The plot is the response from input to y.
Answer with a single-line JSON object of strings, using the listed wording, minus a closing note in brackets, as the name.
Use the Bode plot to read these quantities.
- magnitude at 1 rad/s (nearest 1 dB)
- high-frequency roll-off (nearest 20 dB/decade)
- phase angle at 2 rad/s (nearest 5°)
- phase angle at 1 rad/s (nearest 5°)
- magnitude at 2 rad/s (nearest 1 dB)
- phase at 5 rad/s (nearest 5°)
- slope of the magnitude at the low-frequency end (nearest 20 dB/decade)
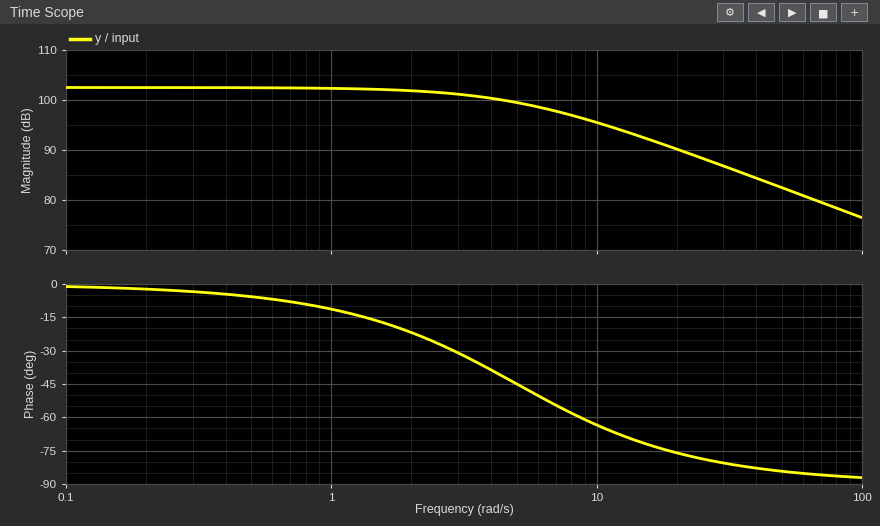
{"magnitude at 1 rad/s": "102 dB", "high-frequency roll-off": "-20 dB/decade", "phase angle at 2 rad/s": "-20°", "phase angle at 1 rad/s": "-10°", "magnitude at 2 rad/s": "102 dB", "phase at 5 rad/s": "-45°", "slope of the magnitude at the low-frequency end": "0 dB/decade"}
